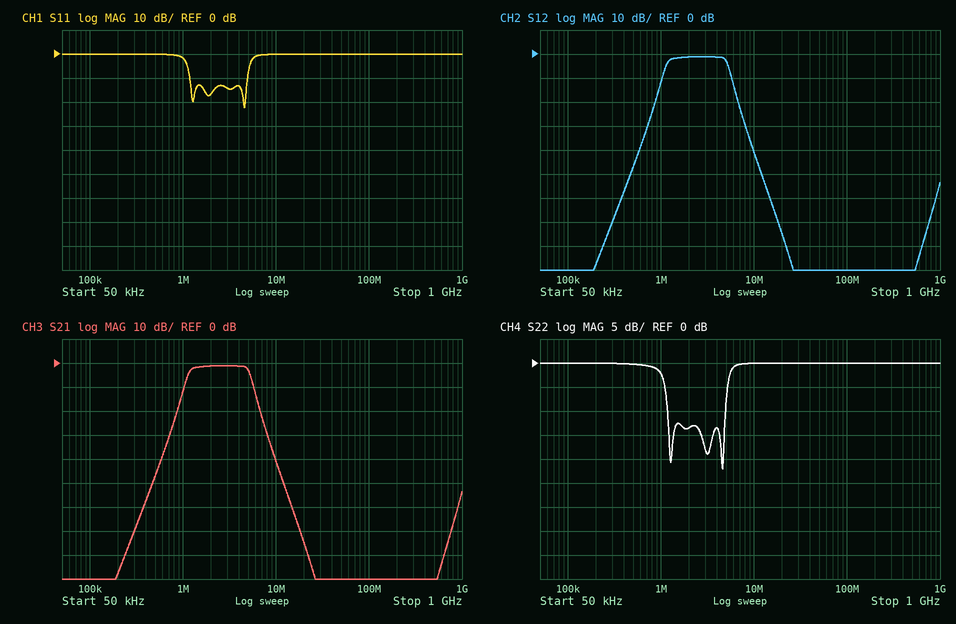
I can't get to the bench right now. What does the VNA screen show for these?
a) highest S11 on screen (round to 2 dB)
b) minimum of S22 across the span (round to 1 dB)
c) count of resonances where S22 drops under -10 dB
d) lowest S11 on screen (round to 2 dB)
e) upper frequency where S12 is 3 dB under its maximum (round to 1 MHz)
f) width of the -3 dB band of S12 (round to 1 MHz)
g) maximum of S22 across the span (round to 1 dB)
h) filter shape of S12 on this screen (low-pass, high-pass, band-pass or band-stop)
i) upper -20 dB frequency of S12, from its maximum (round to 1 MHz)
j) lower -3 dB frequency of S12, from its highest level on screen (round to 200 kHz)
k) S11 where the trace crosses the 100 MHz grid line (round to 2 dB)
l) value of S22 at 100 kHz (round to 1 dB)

0 dB
-22 dB
3
-22 dB
5 MHz
4 MHz
0 dB
band-pass
7 MHz
1.2 MHz
0 dB
0 dB
